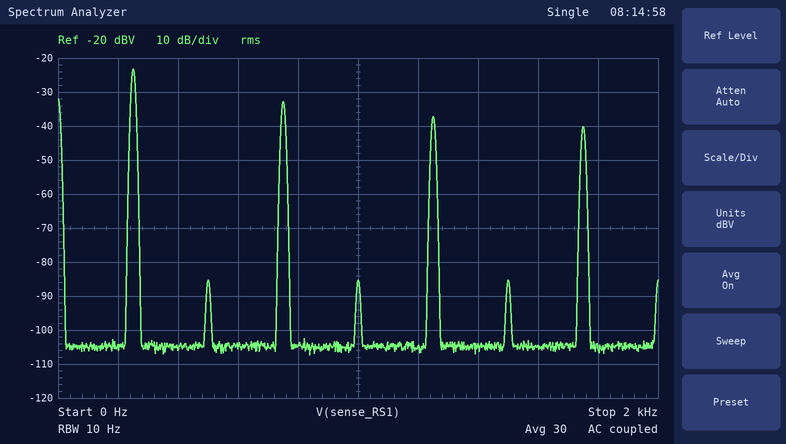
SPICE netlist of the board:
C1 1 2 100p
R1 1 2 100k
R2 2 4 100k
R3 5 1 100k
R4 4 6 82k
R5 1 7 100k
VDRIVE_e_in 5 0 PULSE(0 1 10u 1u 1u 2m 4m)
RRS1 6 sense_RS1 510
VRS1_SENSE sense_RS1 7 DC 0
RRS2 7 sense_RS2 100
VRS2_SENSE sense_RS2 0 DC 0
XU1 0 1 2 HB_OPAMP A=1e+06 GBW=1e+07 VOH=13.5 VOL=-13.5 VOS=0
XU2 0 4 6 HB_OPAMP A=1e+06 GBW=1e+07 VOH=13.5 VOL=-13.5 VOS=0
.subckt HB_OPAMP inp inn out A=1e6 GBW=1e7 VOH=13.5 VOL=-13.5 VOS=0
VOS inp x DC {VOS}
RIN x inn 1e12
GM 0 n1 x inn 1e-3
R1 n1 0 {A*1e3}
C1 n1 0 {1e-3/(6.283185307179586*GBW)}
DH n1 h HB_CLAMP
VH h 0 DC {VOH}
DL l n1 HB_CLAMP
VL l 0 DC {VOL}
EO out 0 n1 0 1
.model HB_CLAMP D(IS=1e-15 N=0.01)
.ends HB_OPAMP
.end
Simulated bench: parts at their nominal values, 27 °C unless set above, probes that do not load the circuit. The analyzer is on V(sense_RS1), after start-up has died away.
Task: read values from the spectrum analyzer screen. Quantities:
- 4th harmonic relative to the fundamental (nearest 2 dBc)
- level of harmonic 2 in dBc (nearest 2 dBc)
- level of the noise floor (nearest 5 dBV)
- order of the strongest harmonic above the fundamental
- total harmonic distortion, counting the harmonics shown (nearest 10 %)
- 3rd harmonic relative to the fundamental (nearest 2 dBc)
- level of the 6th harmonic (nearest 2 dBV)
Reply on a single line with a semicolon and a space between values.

-62 dBc; -62 dBc; -105 dBV; 3; 40 %; -10 dBc; -86 dBV
